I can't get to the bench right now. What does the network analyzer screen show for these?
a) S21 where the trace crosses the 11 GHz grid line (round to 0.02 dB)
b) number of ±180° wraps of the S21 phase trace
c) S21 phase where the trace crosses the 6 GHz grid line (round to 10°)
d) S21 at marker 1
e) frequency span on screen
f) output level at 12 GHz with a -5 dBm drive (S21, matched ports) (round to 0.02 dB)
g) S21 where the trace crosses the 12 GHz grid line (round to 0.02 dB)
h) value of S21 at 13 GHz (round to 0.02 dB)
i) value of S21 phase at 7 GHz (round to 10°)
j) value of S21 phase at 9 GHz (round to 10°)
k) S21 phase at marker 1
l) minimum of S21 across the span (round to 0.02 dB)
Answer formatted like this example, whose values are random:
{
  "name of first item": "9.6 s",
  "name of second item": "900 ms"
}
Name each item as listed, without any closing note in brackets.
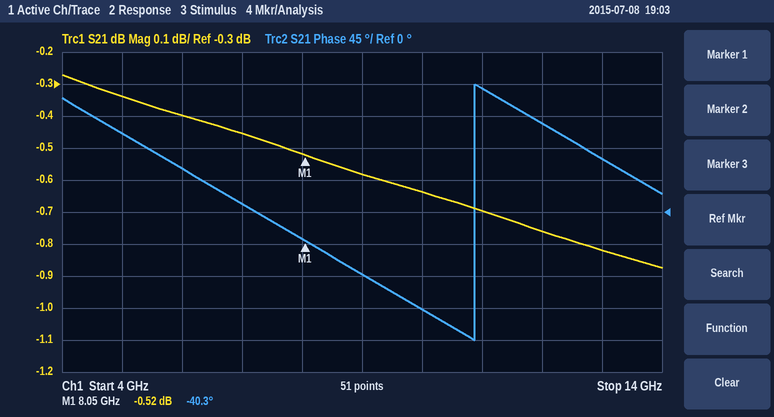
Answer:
{
  "S21 where the trace crosses the 11 GHz grid line": "-0.70 dB",
  "number of ±180° wraps of the S21 phase trace": "1",
  "S21 phase where the trace crosses the 6 GHz grid line": "60°",
  "S21 at marker 1": "-0.52 dB",
  "frequency span on screen": "10 GHz",
  "output level at 12 GHz with a -5 dBm drive (S21, matched ports)": "-5.76 dBm",
  "S21 where the trace crosses the 12 GHz grid line": "-0.76 dB",
  "value of S21 at 13 GHz": "-0.82 dB",
  "value of S21 phase at 7 GHz": "10°",
  "value of S21 phase at 9 GHz": "-90°",
  "S21 phase at marker 1": "-40.3°",
  "minimum of S21 across the span": "-0.88 dB"
}
